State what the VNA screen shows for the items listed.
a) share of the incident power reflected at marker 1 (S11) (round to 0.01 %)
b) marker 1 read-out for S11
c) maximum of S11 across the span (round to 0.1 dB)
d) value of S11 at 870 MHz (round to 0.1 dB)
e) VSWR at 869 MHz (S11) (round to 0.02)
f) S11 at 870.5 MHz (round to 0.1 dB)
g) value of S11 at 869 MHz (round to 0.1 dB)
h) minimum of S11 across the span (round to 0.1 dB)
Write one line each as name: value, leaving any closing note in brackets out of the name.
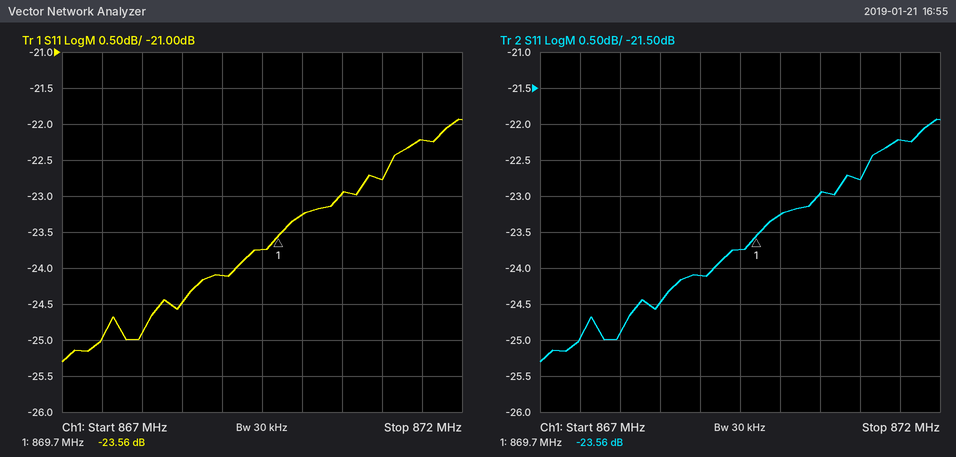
share of the incident power reflected at marker 1 (S11): 0.44 %
marker 1 read-out for S11: -23.56 dB
maximum of S11 across the span: -21.9 dB
value of S11 at 870 MHz: -23.3 dB
VSWR at 869 MHz (S11): 1.14
S11 at 870.5 MHz: -23.0 dB
value of S11 at 869 MHz: -24.1 dB
minimum of S11 across the span: -25.3 dB
